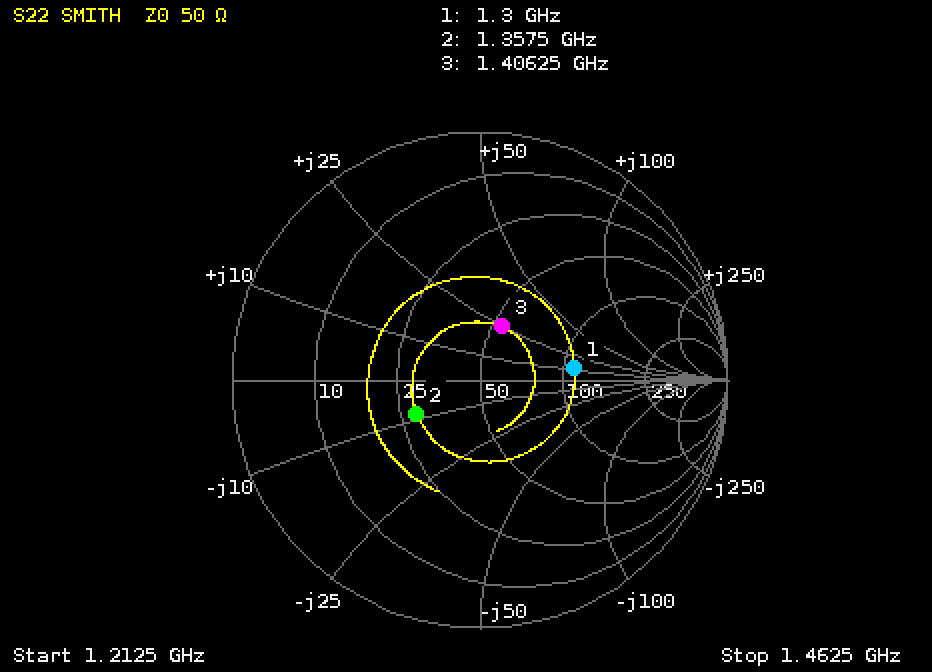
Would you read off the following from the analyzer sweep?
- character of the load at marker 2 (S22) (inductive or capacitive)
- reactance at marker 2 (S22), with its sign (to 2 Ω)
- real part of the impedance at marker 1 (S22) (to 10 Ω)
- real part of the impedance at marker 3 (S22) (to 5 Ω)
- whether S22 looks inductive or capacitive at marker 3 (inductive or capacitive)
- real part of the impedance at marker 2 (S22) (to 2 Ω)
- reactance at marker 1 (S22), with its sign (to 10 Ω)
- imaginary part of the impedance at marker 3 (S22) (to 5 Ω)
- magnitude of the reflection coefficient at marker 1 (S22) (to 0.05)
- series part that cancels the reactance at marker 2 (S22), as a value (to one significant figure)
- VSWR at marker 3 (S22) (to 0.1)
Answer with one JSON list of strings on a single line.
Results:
["capacitive", "-8 Ω", "110 Ω", "55 Ω", "inductive", "28 Ω", "+10 Ω", "+25 Ω", "0.40", "1 nH", "1.6"]
